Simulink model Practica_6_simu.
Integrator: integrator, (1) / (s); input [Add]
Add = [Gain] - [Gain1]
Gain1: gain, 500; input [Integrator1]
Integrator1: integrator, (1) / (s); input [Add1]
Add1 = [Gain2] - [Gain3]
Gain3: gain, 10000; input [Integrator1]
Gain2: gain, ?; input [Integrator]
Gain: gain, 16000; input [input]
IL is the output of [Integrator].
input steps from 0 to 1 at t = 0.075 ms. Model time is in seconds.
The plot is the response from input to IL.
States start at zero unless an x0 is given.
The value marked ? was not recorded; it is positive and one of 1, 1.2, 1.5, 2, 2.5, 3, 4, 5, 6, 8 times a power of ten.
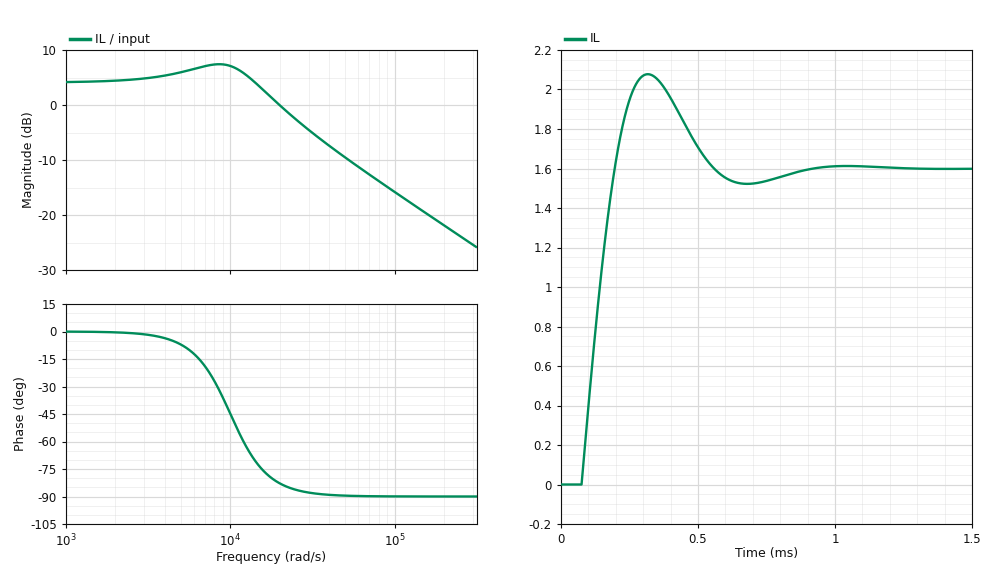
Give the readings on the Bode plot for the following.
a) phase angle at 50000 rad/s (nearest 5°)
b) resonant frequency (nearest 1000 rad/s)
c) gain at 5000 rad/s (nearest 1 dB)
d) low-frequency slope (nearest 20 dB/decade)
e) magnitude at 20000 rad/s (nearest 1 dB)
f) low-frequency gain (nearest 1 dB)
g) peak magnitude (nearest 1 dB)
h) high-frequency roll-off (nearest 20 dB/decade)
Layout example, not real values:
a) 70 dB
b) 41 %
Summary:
a) -90°
b) 8000 rad/s
c) 6 dB
d) 0 dB/decade
e) 0 dB
f) 4 dB
g) 7 dB
h) -20 dB/decade
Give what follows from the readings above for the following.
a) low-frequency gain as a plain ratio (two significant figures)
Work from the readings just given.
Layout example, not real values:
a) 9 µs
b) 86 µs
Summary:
a) 1.6
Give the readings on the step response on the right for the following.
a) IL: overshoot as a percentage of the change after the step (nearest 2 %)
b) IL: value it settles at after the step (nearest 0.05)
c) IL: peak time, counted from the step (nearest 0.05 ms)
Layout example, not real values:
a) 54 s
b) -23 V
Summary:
a) 30 %
b) 1.60
c) 0.25 ms
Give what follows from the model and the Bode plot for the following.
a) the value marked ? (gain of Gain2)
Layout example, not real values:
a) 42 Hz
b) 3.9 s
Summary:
a) 200000
